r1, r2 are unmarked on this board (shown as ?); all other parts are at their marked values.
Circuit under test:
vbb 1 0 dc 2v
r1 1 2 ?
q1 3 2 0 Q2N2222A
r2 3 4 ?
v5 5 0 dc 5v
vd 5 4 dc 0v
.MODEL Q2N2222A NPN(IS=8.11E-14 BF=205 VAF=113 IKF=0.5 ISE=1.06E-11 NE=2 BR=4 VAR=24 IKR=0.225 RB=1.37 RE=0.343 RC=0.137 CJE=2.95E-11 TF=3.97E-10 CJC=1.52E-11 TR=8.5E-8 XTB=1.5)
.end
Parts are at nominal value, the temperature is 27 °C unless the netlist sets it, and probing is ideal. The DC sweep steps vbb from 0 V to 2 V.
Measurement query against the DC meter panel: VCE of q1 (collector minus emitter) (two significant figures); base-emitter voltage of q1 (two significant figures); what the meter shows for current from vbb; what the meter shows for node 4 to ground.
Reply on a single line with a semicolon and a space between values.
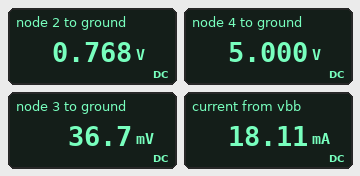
37 mV; 770 mV; 18.11 mA; 5.000 V
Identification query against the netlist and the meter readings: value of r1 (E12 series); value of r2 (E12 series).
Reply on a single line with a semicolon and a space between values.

68 Ω; 180 Ω
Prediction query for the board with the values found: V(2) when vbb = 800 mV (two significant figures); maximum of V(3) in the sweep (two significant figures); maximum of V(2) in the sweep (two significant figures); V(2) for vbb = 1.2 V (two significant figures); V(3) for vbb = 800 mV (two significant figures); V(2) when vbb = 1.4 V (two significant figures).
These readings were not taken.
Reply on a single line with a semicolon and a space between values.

710 mV; 5.0 V; 770 mV; 730 mV; 67 mV; 740 mV
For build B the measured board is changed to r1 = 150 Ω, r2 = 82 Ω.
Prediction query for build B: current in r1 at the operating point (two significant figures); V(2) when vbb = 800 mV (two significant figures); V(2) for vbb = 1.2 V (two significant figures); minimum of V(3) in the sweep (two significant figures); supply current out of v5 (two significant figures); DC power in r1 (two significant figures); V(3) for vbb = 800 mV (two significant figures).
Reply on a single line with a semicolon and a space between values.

8.3 mA; 730 mV; 740 mV; 67 mV; 60 mA; 10 mW; 160 mV
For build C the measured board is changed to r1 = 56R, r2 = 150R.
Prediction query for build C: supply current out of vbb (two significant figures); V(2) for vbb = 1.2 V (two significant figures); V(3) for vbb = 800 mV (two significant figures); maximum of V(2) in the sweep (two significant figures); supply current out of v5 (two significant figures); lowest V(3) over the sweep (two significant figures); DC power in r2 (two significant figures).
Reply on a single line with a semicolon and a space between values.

22 mA; 740 mV; 71 mV; 780 mV; 33 mA; 41 mV; 160 mW
